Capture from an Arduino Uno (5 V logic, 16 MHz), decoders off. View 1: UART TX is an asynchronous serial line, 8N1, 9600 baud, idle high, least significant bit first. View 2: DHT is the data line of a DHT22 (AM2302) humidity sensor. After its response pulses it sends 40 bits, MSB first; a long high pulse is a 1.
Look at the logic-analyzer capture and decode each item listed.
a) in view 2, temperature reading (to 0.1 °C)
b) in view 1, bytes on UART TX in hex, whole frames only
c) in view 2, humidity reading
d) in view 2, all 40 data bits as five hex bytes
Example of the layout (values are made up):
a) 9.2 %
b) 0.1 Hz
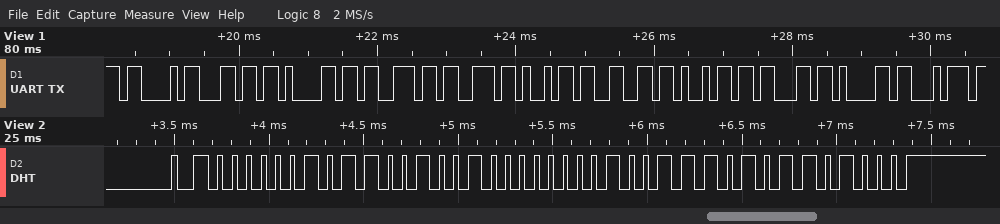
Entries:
a) 15.7 °C
b) 43 6C 61 73 73 69 66 69 63 61 74
c) 71.3 %
d) 02 C9 00 9D 68
